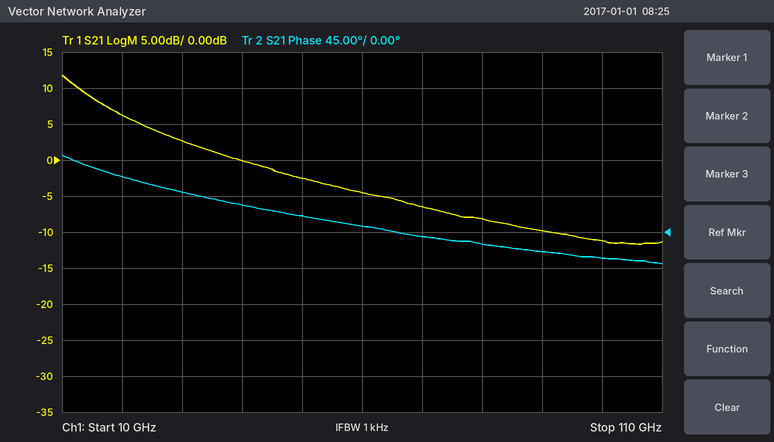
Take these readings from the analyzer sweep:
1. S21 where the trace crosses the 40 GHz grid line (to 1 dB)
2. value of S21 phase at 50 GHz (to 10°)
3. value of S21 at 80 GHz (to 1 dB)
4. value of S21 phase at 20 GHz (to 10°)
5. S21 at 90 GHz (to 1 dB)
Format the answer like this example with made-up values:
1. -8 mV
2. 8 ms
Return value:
1. 0 dB
2. 20°
3. -8 dB
4. 70°
5. -10 dB
